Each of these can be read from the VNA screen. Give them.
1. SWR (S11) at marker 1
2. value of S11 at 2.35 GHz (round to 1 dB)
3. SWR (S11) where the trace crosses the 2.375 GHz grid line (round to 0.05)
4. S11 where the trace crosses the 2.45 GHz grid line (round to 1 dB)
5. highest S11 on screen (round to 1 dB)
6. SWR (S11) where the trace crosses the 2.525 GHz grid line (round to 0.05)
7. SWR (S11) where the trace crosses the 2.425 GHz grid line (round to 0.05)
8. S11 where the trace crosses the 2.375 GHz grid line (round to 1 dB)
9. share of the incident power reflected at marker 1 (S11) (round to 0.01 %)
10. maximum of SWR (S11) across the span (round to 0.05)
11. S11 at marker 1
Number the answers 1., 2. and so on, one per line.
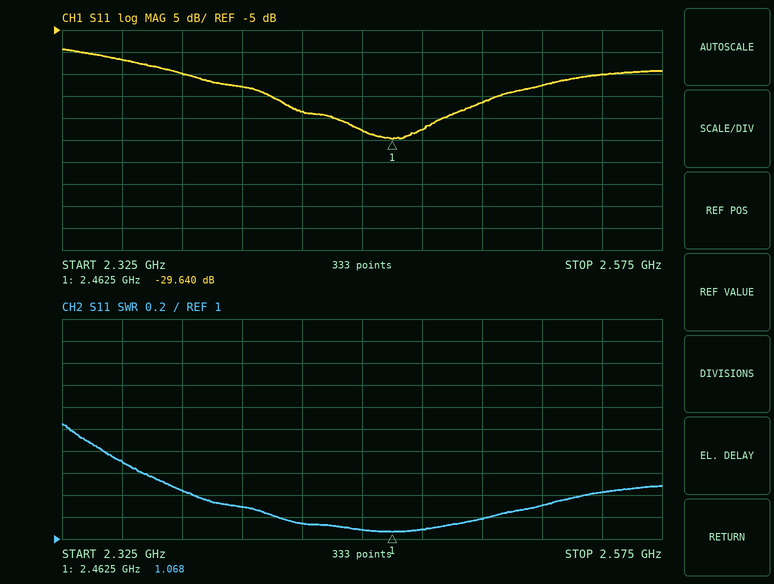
1. 1.068
2. -12 dB
3. 1.45
4. -28 dB
5. -9 dB
6. 1.30
7. 1.15
8. -15 dB
9. 0.11 %
10. 2.05
11. -29.640 dB
